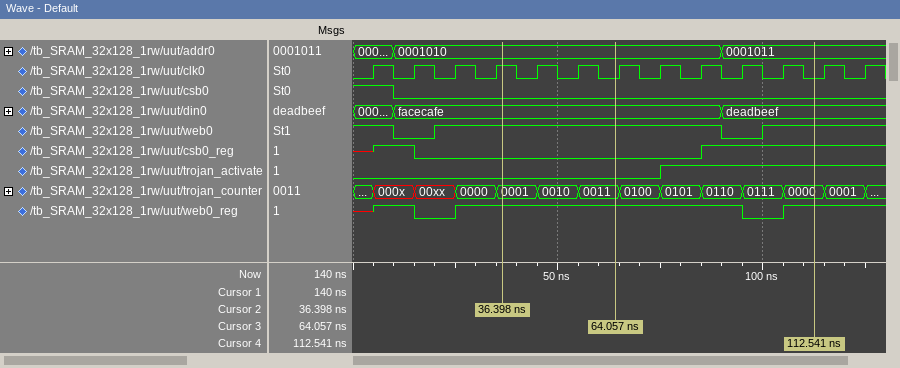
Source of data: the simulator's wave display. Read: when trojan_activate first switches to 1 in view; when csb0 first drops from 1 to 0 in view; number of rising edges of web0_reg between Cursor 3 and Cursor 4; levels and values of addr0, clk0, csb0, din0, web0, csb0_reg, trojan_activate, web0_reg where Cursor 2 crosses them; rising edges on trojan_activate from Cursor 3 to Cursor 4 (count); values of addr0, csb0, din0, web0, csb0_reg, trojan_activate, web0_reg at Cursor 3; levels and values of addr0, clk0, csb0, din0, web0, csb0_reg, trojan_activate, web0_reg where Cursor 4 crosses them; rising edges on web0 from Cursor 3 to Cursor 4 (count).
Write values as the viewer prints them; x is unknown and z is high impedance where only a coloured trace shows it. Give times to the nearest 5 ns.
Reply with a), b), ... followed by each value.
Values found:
a) 75 ns
b) 10 ns
c) 1
d) addr0=0001010, clk0=1, csb0=0, din0=facecafe, web0=1, csb0_reg=0, trojan_activate=0, web0_reg=1
e) 1
f) addr0=0001010, csb0=0, din0=facecafe, web0=1, csb0_reg=0, trojan_activate=0, web0_reg=1
g) addr0=0001011, clk0=0, csb0=0, din0=deadbeef, web0=1, csb0_reg=1, trojan_activate=1, web0_reg=1
h) 1
